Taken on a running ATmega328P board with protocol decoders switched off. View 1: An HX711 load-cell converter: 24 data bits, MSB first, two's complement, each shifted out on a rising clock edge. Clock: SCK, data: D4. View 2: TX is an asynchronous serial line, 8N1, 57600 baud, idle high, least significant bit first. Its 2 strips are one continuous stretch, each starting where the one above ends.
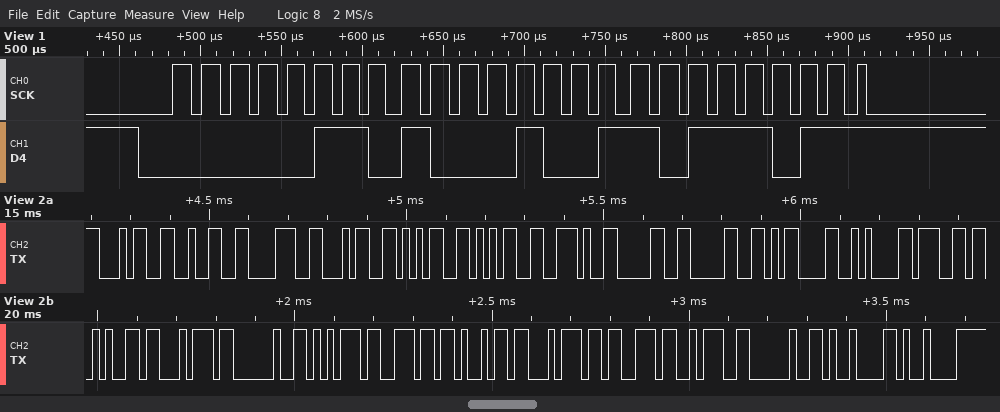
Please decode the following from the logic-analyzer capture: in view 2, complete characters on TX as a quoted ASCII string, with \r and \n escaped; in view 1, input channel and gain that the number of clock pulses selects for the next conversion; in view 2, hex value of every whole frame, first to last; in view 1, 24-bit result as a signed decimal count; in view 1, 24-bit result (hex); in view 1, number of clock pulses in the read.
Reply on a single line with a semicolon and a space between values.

"428455.00\r\nget units: \t\t"; channel A, gain 128; 34 32 38 34 35 35 2E 30 30 0D 0A 67 65 74 20 75 6E 69 74 73 3A 20 09 09; 428475; 0x0689BB; 25
